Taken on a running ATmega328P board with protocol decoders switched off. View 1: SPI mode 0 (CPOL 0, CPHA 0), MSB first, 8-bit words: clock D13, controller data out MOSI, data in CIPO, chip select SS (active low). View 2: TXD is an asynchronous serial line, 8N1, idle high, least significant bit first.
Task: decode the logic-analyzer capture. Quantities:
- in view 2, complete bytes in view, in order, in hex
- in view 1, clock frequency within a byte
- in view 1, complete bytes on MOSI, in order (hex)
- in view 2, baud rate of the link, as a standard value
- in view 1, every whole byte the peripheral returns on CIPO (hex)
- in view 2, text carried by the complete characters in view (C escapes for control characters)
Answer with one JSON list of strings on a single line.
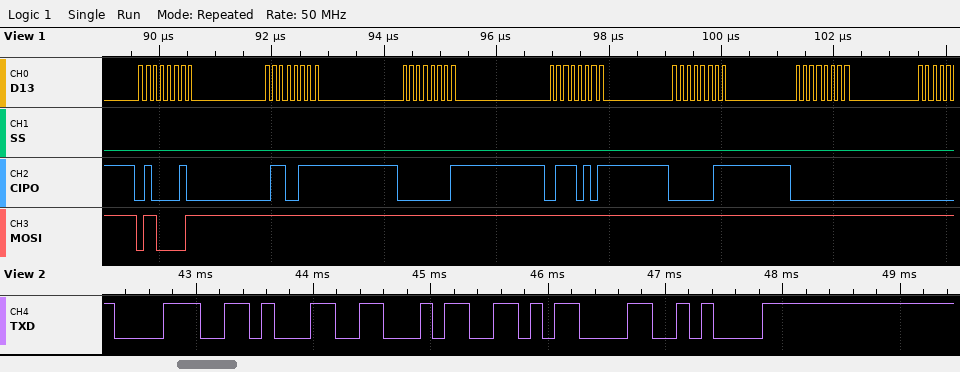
["0x38 0x31 0x34 0x0D 0x0A", "8 MHz", "61 FF FF FF FF FF", "9600 baud", "42 67 01 75 03 00", "\"814\\r\\n\""]
